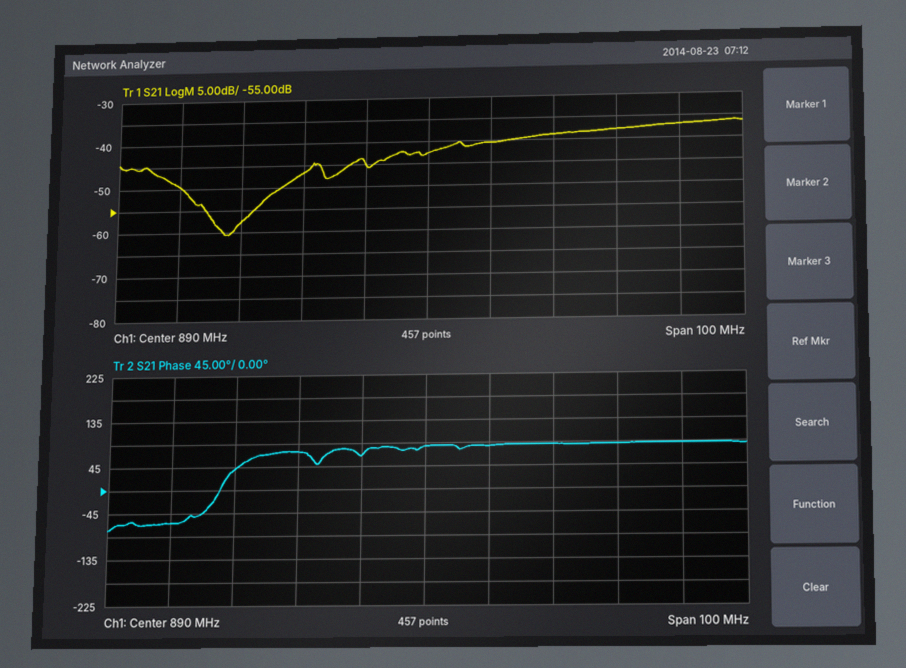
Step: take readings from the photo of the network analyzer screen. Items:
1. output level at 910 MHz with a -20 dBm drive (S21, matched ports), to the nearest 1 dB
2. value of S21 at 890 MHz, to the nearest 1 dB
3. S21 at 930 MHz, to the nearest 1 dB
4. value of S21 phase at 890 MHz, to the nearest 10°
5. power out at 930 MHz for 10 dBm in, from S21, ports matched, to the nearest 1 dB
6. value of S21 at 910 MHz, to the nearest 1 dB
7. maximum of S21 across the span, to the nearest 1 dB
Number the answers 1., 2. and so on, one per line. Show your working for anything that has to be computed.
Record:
1. -20 dBm + (-39 dB) = -59 dBm
2. -43 dB
3. -37 dB
4. 80°
5. 10 dBm + (-37 dB) = -27 dBm
6. -39 dB
7. -36 dB
